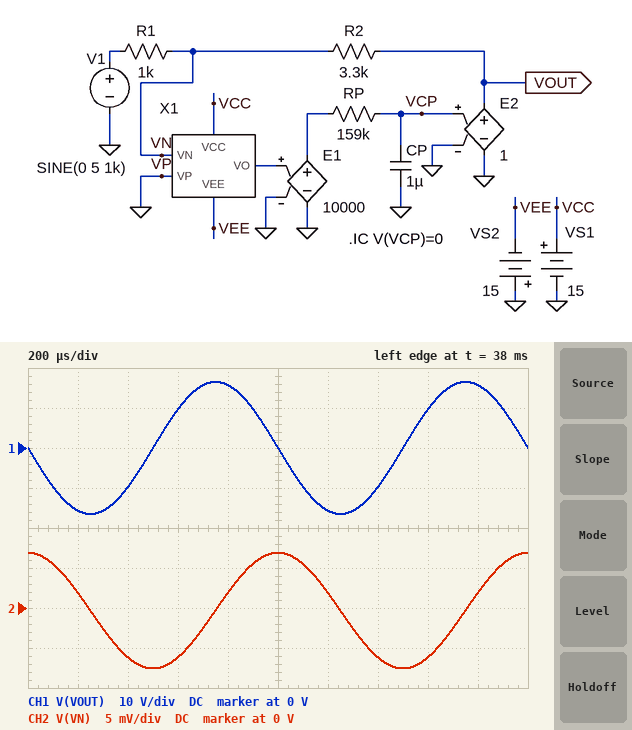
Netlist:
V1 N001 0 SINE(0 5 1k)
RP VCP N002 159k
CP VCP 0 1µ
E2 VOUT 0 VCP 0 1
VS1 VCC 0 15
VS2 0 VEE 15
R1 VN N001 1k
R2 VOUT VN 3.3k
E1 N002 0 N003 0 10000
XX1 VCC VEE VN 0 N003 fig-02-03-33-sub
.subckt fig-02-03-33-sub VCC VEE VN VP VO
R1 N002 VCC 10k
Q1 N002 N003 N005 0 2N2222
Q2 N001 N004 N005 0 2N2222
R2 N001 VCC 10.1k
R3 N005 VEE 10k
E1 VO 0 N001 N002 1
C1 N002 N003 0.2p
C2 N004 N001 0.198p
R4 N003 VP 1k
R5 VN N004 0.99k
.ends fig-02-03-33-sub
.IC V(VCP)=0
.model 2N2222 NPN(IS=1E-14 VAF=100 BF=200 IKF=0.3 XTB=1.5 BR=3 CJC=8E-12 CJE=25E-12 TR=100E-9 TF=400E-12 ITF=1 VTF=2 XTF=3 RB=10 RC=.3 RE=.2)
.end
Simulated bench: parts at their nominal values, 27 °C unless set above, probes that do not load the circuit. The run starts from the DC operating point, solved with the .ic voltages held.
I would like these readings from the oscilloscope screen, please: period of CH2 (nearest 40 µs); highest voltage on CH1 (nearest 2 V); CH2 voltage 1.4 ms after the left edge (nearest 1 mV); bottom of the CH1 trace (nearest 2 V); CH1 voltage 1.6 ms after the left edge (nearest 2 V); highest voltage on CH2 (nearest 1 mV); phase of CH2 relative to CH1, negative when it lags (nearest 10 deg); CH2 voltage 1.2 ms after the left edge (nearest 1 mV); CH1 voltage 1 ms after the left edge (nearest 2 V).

1.00 ms
16 V
-6 mV
-16 V
10 V
7 mV
-90 deg
2 mV
0 V
